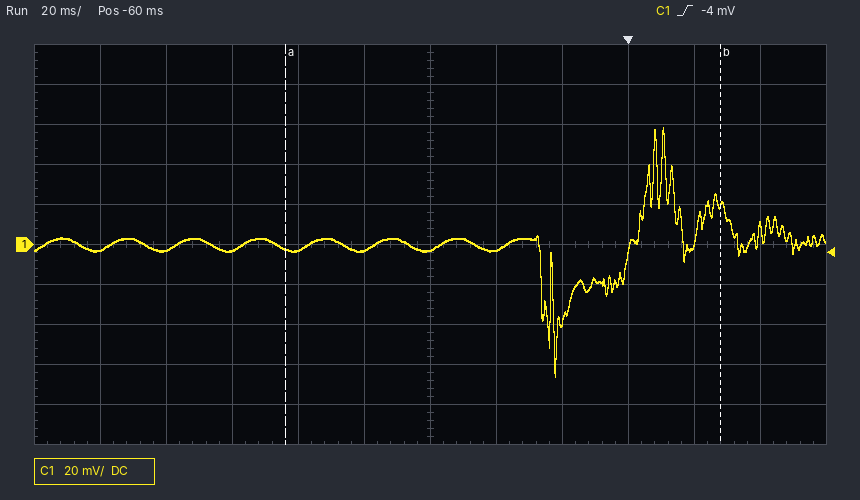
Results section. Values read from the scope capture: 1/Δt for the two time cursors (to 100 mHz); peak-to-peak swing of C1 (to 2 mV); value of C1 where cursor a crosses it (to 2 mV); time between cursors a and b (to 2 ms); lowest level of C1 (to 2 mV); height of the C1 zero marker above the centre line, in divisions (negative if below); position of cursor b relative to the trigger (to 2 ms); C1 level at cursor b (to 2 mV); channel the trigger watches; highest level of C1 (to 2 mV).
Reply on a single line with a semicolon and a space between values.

7.6 Hz; 124 mV; -2 mV; 132 ms; -66 mV; 0.0 div; +28 ms; 20 mV; C1; 58 mV
